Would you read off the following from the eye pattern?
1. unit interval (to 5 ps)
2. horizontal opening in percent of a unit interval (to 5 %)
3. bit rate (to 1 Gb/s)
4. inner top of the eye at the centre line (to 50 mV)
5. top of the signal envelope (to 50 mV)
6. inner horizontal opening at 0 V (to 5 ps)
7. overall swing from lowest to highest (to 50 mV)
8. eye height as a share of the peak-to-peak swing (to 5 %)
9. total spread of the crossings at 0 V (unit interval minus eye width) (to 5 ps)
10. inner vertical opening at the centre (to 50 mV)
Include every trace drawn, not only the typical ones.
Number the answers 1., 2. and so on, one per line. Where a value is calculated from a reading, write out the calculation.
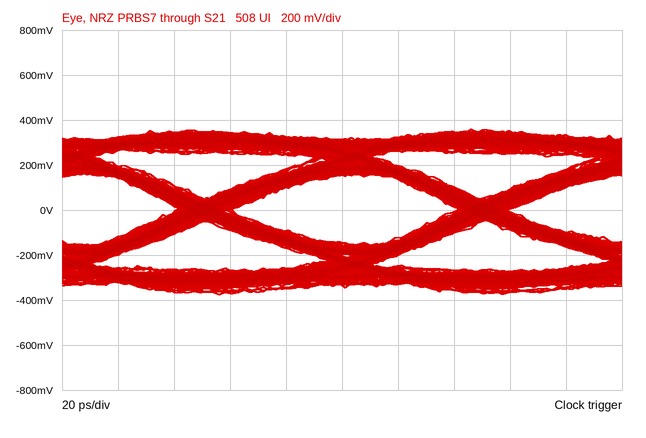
1. 100 ps
2. 80 ps / 100 ps ≈ 80 %
3. 10 Gb/s
4. 150 mV
5. 350 mV
6. 80 ps
7. 750 mV
8. 300 mV / 750 mV ≈ 40 %
9. 20 ps
10. 300 mV
